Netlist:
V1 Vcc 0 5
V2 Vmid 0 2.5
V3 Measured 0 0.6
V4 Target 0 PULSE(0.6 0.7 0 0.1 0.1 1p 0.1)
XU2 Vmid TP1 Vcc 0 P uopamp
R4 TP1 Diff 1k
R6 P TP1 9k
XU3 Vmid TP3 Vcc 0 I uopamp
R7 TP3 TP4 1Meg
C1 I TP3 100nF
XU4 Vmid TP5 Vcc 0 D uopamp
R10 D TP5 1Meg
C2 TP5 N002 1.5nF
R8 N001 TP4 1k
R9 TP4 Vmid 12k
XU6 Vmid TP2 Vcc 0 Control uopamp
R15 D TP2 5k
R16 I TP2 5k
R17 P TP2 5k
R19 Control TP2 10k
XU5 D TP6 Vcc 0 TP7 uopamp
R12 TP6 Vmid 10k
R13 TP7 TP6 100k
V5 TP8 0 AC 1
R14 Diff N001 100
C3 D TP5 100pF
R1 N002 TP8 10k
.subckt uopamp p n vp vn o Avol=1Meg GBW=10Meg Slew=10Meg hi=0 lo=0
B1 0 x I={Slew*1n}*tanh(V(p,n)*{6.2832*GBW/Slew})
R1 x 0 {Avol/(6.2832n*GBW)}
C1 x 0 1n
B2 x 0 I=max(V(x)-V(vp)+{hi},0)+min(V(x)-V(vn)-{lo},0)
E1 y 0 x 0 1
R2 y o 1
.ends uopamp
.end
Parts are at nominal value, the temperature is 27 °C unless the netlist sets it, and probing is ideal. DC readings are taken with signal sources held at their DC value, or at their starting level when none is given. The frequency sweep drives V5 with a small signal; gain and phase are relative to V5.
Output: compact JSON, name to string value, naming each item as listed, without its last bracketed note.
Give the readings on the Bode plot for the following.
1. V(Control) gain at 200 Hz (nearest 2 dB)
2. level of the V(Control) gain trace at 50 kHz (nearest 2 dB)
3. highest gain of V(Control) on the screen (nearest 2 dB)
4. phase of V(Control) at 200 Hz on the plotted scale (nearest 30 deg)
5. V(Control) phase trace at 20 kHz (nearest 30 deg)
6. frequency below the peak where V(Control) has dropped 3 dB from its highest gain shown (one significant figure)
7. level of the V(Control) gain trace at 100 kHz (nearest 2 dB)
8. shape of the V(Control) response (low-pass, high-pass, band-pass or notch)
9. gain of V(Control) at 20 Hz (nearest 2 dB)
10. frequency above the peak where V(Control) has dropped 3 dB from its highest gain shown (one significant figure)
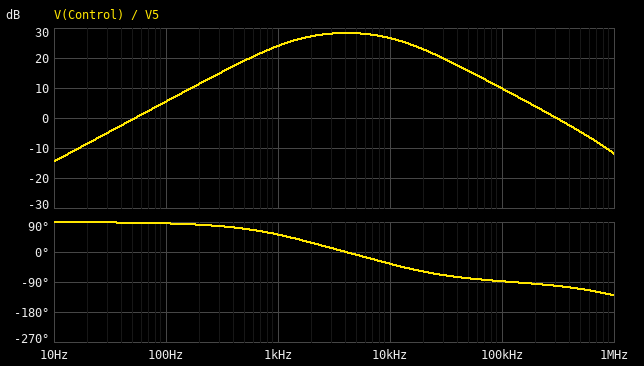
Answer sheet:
{"V(Control) gain at 200 Hz": "12 dB", "level of the V(Control) gain trace at 50 kHz": "16 dB", "highest gain of V(Control) on the screen": "28 dB", "phase of V(Control) at 200 Hz on the plotted scale": "90 deg", "V(Control) phase trace at 20 kHz": "-60 deg", "frequency below the peak where V(Control) has dropped 3 dB from its highest gain shown": "1 kHz", "level of the V(Control) gain trace at 100 kHz": "10 dB", "shape of the V(Control) response": "band-pass", "gain of V(Control) at 20 Hz": "-8 dB", "frequency above the peak where V(Control) has dropped 3 dB from its highest gain shown": "10 kHz"}
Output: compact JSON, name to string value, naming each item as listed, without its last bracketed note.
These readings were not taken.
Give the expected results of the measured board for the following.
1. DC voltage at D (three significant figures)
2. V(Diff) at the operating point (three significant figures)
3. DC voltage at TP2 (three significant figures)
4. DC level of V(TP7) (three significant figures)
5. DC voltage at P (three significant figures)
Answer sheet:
{"DC voltage at D": "2.50 V", "V(Diff) at the operating point": "2.50 V", "DC voltage at TP2": "2.50 V", "DC level of V(TP7)": "2.50 V", "DC voltage at P": "2.50 V"}
